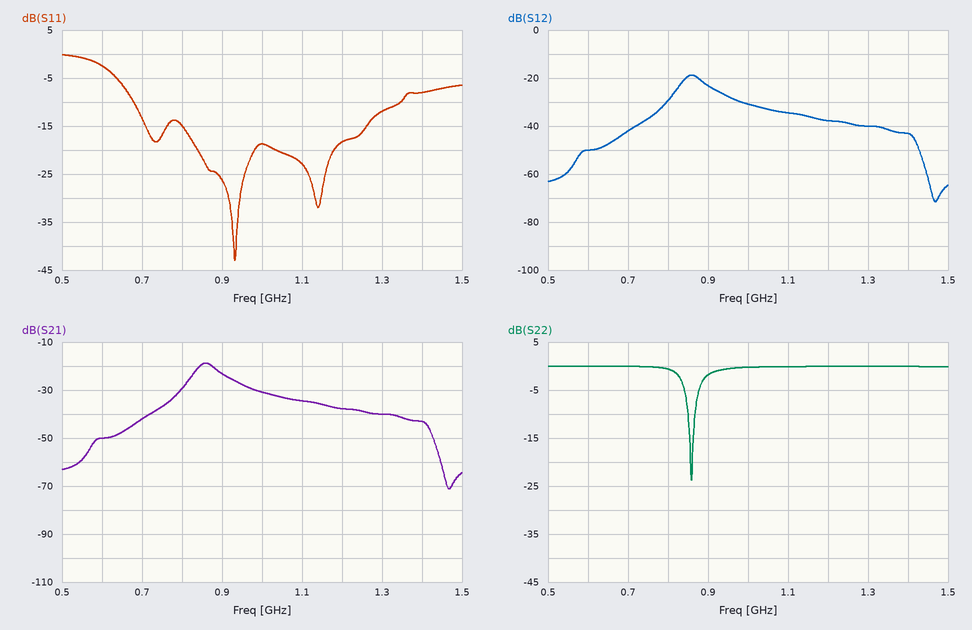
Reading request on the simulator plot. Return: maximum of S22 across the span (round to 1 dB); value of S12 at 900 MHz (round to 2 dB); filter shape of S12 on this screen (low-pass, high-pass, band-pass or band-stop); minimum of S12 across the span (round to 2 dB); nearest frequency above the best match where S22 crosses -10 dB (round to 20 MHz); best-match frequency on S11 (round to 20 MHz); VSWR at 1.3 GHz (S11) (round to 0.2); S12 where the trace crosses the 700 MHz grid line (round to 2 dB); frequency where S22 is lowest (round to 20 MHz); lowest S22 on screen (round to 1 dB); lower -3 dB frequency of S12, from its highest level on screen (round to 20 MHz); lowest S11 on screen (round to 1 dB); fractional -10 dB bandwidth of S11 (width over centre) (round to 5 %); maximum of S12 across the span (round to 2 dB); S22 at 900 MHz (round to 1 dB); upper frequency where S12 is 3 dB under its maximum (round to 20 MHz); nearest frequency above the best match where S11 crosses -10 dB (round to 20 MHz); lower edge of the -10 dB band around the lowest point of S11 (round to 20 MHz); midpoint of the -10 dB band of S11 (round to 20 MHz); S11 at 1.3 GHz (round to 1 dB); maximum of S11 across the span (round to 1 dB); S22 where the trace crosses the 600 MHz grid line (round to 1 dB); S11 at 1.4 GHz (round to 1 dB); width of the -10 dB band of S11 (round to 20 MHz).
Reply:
0 dB
-24 dB
band-pass
-72 dB
860 MHz
940 MHz
1.6
-42 dB
860 MHz
-24 dB
840 MHz
-43 dB
65 %
-18 dB
-2 dB
880 MHz
1.34 GHz
680 MHz
1.02 GHz
-12 dB
0 dB
0 dB
-8 dB
660 MHz
